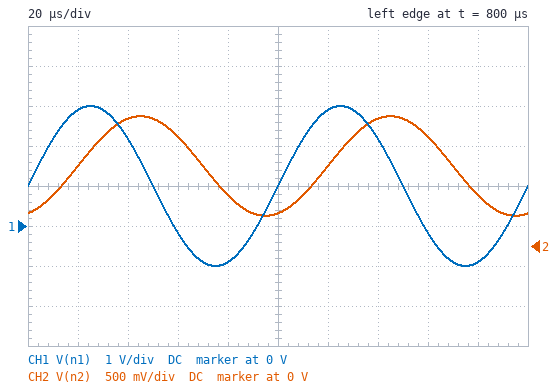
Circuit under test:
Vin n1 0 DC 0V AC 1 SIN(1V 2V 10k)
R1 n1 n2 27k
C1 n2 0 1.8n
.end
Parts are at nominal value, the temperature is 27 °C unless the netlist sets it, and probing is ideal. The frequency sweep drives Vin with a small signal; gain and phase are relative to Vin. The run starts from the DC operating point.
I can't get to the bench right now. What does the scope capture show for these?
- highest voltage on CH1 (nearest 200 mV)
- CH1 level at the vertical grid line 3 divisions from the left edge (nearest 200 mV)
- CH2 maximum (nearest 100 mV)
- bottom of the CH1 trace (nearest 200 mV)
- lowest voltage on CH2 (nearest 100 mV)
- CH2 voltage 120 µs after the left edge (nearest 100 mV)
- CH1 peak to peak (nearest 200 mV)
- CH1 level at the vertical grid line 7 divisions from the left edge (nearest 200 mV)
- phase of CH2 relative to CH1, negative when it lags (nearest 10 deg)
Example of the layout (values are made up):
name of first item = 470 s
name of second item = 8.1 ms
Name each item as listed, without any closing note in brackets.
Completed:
highest voltage on CH1 = 3.0 V
CH1 level at the vertical grid line 3 divisions from the left edge = -200 mV
CH2 maximum = 1.6 V
bottom of the CH1 trace = -1.0 V
lowest voltage on CH2 = 400 mV
CH2 voltage 120 µs after the left edge = 1.0 V
CH1 peak to peak = 4.0 V
CH1 level at the vertical grid line 7 divisions from the left edge = 2.2 V
phase of CH2 relative to CH1, negative when it lags = -70 deg
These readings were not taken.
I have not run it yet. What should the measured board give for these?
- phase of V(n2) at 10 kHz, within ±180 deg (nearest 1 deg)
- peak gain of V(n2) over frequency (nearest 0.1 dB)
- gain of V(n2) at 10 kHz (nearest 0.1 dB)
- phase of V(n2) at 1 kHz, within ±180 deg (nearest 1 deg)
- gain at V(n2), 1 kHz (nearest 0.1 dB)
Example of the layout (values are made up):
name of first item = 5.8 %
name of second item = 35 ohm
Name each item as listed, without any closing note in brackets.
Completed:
phase of V(n2) at 10 kHz, within ±180 deg = -72 deg
peak gain of V(n2) over frequency = 0 dB
gain of V(n2) at 10 kHz = -10.1 dB
phase of V(n2) at 1 kHz, within ±180 deg = -17 deg
gain at V(n2), 1 kHz = -0.4 dB
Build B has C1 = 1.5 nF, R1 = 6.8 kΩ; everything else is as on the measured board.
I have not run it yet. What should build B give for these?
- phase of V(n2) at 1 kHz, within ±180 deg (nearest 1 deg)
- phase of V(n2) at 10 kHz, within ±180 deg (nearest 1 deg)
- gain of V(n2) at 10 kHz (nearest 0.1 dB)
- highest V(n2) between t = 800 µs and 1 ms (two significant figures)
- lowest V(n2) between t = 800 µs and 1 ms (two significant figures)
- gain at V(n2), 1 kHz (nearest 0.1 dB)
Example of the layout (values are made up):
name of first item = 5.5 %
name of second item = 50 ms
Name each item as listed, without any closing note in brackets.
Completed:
phase of V(n2) at 1 kHz, within ±180 deg = -4 deg
phase of V(n2) at 10 kHz, within ±180 deg = -33 deg
gain of V(n2) at 10 kHz = -1.5 dB
highest V(n2) between t = 800 µs and 1 ms = 2.7 V
lowest V(n2) between t = 800 µs and 1 ms = -680 mV
gain at V(n2), 1 kHz = 0 dB
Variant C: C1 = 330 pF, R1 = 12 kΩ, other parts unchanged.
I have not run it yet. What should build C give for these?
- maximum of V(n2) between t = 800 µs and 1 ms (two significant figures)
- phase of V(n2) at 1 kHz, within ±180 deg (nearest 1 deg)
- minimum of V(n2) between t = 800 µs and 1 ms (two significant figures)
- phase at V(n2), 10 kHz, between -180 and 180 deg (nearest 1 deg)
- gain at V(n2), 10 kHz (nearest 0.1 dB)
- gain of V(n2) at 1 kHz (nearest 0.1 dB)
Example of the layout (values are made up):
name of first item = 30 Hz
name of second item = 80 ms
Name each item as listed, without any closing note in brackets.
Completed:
maximum of V(n2) between t = 800 µs and 1 ms = 2.9 V
phase of V(n2) at 1 kHz, within ±180 deg = -1 deg
minimum of V(n2) between t = 800 µs and 1 ms = -940 mV
phase at V(n2), 10 kHz, between -180 and 180 deg = -14 deg
gain at V(n2), 10 kHz = -0.3 dB
gain of V(n2) at 1 kHz = 0 dB
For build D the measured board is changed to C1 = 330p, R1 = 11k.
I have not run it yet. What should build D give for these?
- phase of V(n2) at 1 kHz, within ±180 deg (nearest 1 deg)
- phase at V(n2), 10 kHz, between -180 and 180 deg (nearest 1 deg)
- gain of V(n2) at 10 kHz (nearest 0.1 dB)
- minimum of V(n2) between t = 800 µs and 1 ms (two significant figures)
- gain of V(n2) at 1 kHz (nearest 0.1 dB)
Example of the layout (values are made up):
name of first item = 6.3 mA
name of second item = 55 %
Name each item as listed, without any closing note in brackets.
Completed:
phase of V(n2) at 1 kHz, within ±180 deg = -1 deg
phase at V(n2), 10 kHz, between -180 and 180 deg = -13 deg
gain of V(n2) at 10 kHz = -0.2 dB
minimum of V(n2) between t = 800 µs and 1 ms = -950 mV
gain of V(n2) at 1 kHz = 0 dB
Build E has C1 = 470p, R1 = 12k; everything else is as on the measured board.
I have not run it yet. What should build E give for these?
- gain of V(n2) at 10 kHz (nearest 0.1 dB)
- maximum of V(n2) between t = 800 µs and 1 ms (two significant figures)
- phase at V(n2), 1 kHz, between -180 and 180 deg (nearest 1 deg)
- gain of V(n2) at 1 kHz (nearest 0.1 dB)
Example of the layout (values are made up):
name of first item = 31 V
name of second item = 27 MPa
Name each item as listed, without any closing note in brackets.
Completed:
gain of V(n2) at 10 kHz = -0.5 dB
maximum of V(n2) between t = 800 µs and 1 ms = 2.9 V
phase at V(n2), 1 kHz, between -180 and 180 deg = -2 deg
gain of V(n2) at 1 kHz = 0 dB
